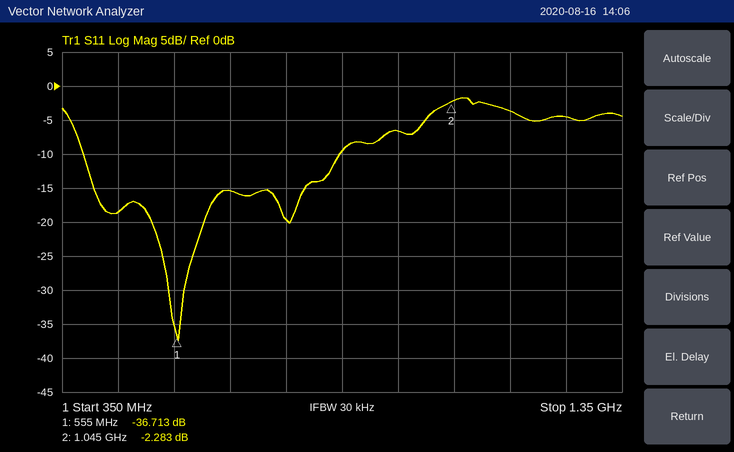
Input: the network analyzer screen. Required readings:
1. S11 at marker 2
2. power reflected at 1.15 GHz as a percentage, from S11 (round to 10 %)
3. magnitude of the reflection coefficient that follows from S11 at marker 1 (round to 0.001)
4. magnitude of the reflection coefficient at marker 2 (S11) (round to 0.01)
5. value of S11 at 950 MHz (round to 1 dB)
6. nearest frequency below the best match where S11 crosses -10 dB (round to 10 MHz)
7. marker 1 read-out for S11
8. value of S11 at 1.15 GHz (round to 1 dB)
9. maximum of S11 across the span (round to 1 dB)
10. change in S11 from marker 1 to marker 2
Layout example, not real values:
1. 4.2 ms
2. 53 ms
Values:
1. -2.283 dB
2. 40 %
3. 0.015
4. 0.77
5. -7 dB
6. 390 MHz
7. -36.713 dB
8. -4 dB
9. -2 dB
10. 34.430 dB
